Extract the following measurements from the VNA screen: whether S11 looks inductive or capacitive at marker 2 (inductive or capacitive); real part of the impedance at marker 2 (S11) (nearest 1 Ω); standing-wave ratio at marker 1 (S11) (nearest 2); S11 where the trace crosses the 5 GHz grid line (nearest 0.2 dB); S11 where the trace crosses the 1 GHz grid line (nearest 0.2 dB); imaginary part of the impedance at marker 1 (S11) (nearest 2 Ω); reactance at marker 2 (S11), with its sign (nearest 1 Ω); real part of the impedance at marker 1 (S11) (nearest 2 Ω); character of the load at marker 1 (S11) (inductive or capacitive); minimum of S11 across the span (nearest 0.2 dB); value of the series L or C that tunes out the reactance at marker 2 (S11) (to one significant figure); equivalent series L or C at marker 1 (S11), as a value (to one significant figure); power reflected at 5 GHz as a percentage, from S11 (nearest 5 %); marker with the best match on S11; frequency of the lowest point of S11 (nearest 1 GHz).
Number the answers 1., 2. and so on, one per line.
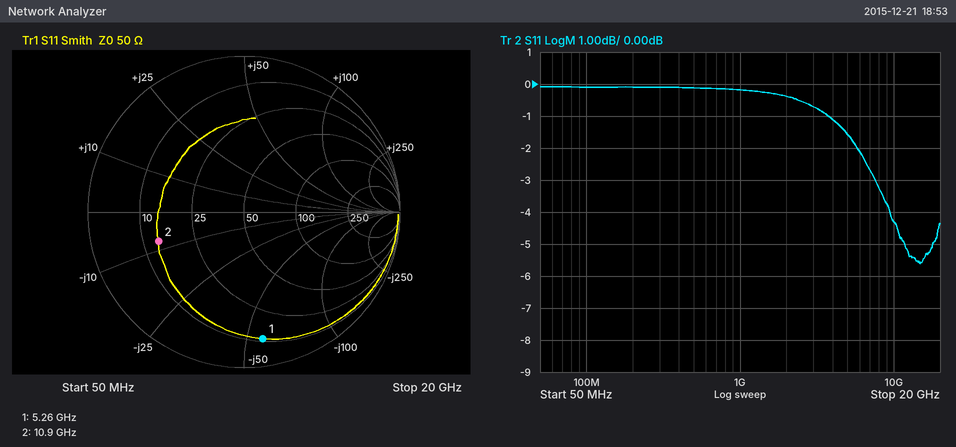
1. capacitive
2. 14 Ω
3. 10
4. -1.6 dB
5. -0.2 dB
6. -56 Ω
7. -8 Ω
8. 12 Ω
9. capacitive
10. -5.6 dB
11. 100 pH
12. 500 fF
13. 70 %
14. marker 2
15. 15 GHz
